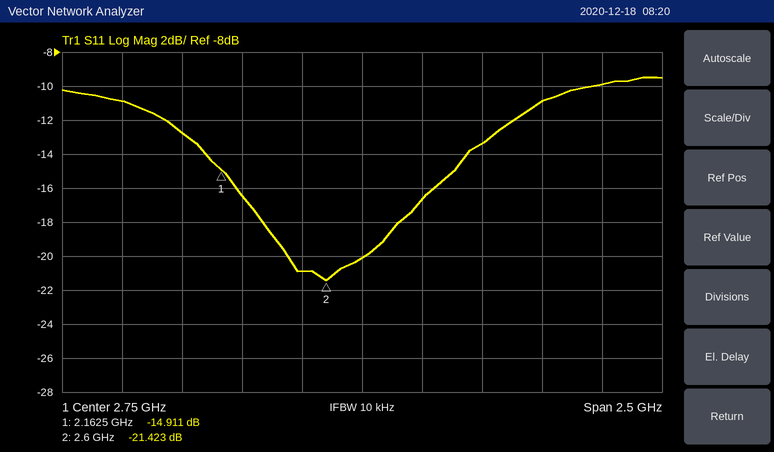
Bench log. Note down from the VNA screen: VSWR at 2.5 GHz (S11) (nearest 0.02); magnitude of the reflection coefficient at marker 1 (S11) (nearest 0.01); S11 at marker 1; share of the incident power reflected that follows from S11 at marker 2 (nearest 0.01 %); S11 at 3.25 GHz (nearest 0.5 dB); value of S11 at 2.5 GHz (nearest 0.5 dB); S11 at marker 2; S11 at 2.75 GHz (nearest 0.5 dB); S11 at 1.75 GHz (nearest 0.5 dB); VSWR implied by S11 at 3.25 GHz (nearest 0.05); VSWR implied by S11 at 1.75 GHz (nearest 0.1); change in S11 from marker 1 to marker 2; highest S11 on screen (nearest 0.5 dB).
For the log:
1.20
0.18
-14.911 dB
0.72 %
-13.5 dB
-21.0 dB
-21.423 dB
-20.0 dB
-11.0 dB
1.55
1.8
-6.512 dB
-9.5 dB
